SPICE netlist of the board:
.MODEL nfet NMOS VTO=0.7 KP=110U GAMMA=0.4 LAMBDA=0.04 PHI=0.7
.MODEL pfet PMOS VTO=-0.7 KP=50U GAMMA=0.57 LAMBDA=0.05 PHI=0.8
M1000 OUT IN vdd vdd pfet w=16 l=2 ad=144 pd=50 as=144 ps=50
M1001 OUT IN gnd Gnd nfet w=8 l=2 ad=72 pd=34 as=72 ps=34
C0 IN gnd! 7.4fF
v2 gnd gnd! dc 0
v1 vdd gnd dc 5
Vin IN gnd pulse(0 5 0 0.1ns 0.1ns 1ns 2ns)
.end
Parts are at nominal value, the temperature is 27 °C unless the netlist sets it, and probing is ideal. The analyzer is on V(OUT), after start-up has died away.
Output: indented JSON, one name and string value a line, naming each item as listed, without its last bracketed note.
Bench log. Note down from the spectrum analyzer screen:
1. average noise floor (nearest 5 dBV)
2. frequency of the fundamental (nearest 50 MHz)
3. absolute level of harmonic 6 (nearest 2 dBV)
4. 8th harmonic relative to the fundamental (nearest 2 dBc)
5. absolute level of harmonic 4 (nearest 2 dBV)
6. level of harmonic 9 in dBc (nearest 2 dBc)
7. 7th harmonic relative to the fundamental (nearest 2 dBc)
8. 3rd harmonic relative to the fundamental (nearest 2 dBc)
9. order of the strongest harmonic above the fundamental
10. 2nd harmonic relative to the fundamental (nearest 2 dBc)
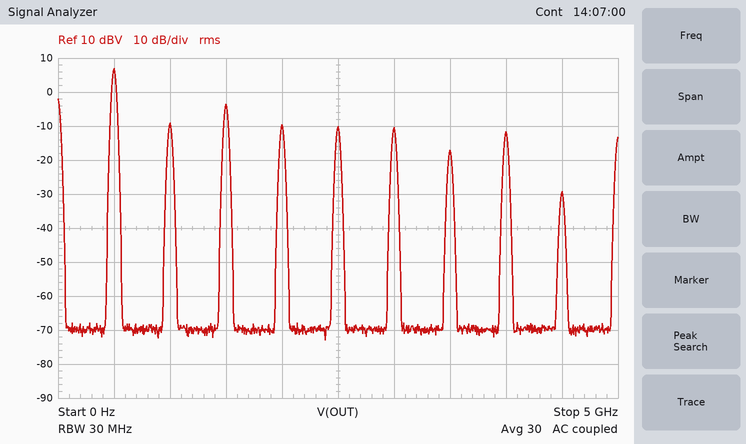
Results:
{
  "average noise floor": "-70 dBV",
  "frequency of the fundamental": "500 MHz",
  "absolute level of harmonic 6": "-10 dBV",
  "8th harmonic relative to the fundamental": "-18 dBc",
  "absolute level of harmonic 4": "-10 dBV",
  "level of harmonic 9 in dBc": "-36 dBc",
  "7th harmonic relative to the fundamental": "-24 dBc",
  "3rd harmonic relative to the fundamental": "-10 dBc",
  "order of the strongest harmonic above the fundamental": "3",
  "2nd harmonic relative to the fundamental": "-16 dBc"
}
